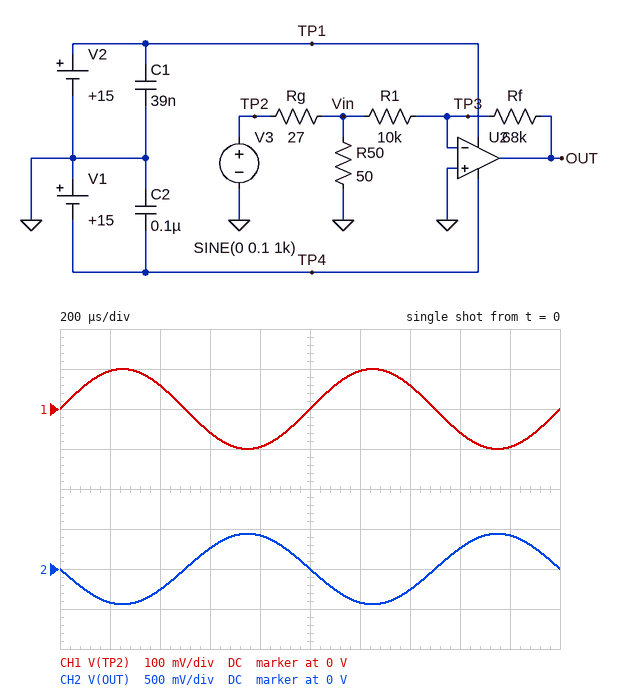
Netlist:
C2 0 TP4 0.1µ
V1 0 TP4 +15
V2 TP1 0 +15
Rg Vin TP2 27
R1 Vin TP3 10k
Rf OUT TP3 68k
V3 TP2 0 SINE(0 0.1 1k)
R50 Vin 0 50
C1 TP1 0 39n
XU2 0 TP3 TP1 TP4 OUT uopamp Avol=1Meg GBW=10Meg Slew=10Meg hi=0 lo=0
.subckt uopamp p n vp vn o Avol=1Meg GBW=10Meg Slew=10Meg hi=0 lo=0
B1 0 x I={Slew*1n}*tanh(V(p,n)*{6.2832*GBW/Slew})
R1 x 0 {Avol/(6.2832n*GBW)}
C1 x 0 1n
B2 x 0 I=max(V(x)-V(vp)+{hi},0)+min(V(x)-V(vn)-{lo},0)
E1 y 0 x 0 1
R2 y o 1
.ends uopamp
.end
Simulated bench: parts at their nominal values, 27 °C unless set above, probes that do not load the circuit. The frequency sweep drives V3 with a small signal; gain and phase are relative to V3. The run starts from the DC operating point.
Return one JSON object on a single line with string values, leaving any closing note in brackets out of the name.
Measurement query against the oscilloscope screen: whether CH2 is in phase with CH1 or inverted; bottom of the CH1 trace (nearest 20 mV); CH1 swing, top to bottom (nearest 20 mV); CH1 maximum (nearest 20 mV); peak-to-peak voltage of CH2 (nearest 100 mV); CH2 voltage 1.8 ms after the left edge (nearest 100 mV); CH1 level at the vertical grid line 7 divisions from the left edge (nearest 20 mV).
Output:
{"whether CH2 is in phase with CH1 or inverted": "inverted", "bottom of the CH1 trace": "-100 mV", "CH1 swing, top to bottom": "200 mV", "CH1 maximum": "100 mV", "peak-to-peak voltage of CH2": "900 mV", "CH2 voltage 1.8 ms after the left edge": "400 mV", "CH1 level at the vertical grid line 7 divisions from the left edge": "60 mV"}
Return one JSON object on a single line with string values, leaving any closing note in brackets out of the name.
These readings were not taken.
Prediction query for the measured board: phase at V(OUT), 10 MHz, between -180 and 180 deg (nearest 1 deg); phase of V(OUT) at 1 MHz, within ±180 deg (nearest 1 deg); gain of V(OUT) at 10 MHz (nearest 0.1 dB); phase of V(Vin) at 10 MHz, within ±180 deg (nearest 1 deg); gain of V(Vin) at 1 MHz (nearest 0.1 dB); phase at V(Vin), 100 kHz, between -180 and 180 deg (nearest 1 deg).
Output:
{"phase at V(OUT), 10 MHz, between -180 and 180 deg": "97 deg", "phase of V(OUT) at 1 MHz, within ±180 deg": "142 deg", "gain of V(OUT) at 10 MHz": "-5.0 dB", "phase of V(Vin) at 10 MHz, within ±180 deg": "0 deg", "gain of V(Vin) at 1 MHz": "-3.8 dB", "phase at V(Vin), 100 kHz, between -180 and 180 deg": "0 deg"}
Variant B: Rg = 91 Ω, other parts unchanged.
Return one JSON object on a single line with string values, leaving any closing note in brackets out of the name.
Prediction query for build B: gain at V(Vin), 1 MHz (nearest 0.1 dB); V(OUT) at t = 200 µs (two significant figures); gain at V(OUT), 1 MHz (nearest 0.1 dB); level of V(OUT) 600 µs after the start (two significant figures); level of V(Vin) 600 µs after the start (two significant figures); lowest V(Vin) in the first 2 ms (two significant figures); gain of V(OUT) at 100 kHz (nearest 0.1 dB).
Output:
{"gain at V(Vin), 1 MHz": "-9.0 dB", "V(OUT) at t = 200 µs": "-230 mV", "gain at V(OUT), 1 MHz": "5.6 dB", "level of V(OUT) 600 µs after the start": "140 mV", "level of V(Vin) 600 µs after the start": "-21 mV", "lowest V(Vin) in the first 2 ms": "-35 mV", "gain of V(OUT) at 100 kHz": "7.6 dB"}
